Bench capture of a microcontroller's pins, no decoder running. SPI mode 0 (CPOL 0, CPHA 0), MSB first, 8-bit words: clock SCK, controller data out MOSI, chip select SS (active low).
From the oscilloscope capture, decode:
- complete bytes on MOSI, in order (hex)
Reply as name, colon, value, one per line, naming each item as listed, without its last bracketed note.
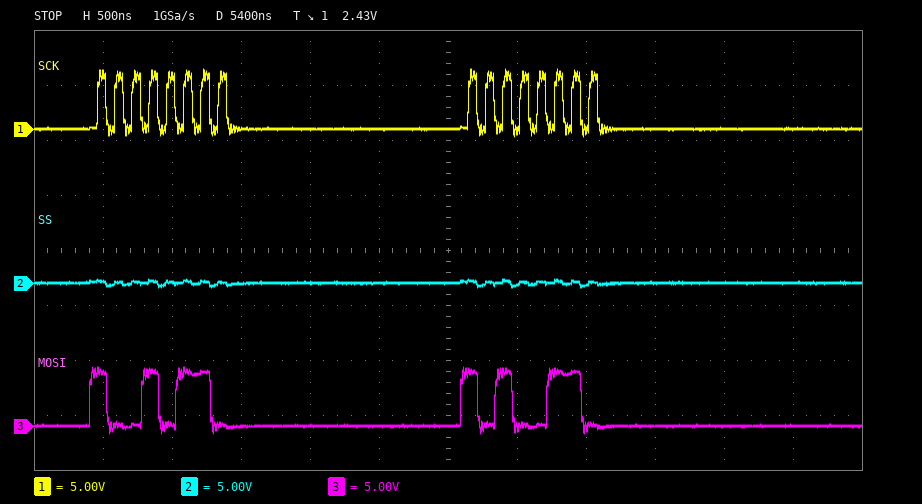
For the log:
complete bytes on MOSI, in order: 0x96 0xA6
